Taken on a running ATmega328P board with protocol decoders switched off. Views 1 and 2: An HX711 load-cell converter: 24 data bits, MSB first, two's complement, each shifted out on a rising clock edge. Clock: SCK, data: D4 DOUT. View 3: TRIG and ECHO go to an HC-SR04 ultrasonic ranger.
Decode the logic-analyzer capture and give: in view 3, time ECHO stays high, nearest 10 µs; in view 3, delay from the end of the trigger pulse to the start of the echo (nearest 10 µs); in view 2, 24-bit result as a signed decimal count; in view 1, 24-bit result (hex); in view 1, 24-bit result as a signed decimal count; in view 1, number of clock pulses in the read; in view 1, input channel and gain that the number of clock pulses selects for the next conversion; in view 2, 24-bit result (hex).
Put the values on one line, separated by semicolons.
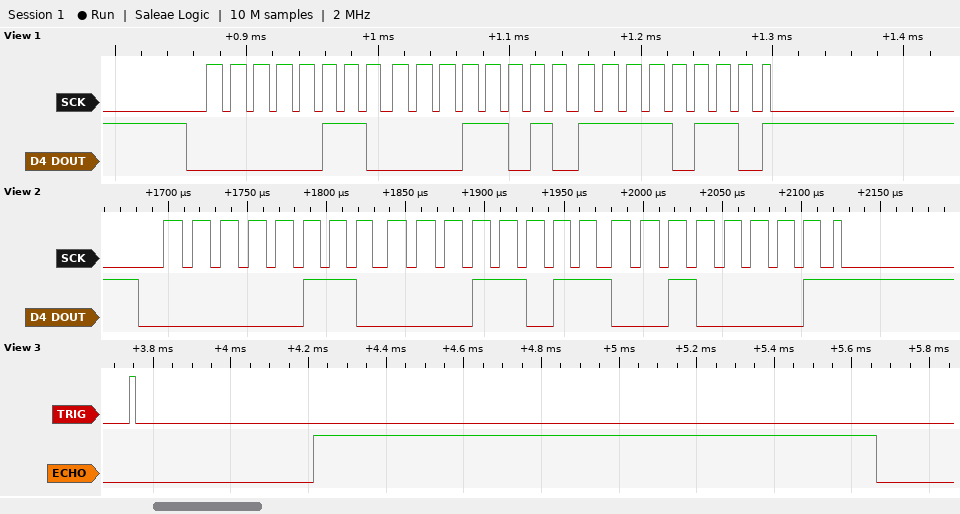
1450 µs; 460 µs; 400161; 0x061AF6; 400118; 25; channel A, gain 128; 0x061B21
